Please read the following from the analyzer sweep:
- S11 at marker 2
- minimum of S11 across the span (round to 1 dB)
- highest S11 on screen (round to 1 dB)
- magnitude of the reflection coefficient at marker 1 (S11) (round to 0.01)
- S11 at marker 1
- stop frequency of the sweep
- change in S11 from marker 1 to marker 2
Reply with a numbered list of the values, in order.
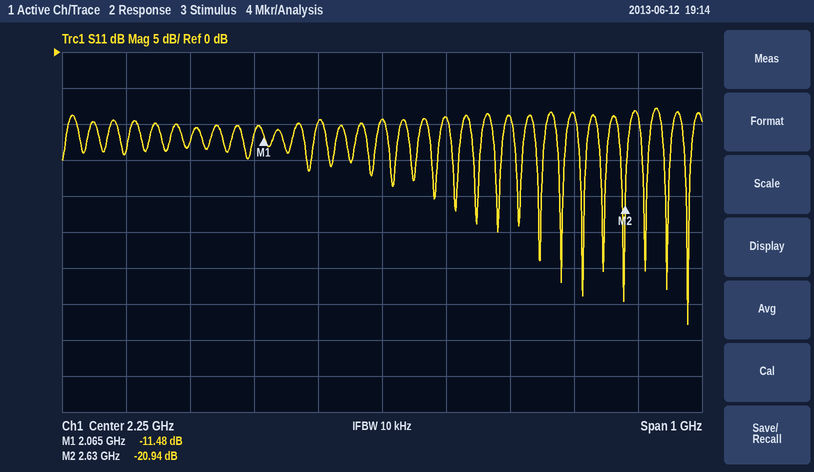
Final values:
1. -20.94 dB
2. -38 dB
3. -8 dB
4. 0.27
5. -11.48 dB
6. 2.75 GHz
7. -9.46 dB
